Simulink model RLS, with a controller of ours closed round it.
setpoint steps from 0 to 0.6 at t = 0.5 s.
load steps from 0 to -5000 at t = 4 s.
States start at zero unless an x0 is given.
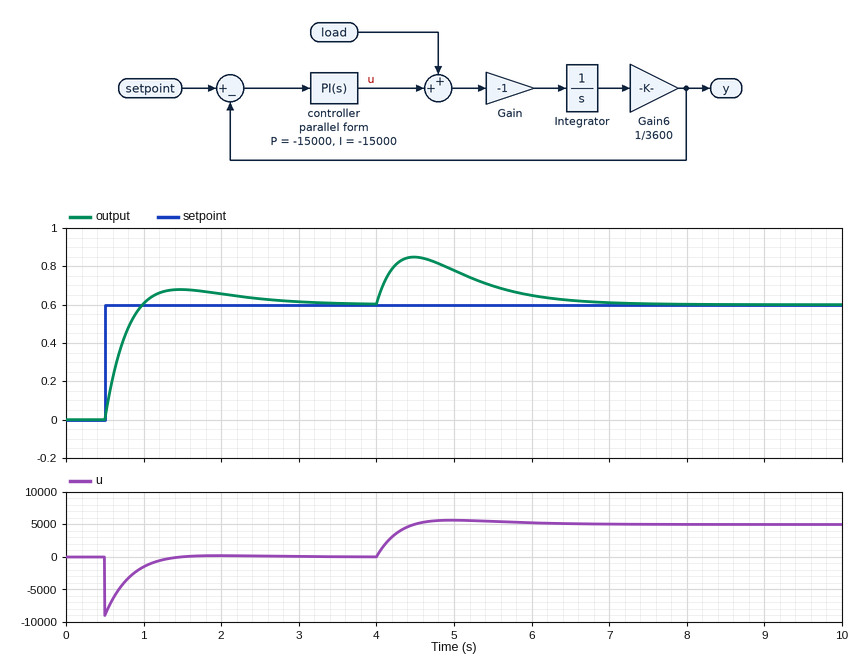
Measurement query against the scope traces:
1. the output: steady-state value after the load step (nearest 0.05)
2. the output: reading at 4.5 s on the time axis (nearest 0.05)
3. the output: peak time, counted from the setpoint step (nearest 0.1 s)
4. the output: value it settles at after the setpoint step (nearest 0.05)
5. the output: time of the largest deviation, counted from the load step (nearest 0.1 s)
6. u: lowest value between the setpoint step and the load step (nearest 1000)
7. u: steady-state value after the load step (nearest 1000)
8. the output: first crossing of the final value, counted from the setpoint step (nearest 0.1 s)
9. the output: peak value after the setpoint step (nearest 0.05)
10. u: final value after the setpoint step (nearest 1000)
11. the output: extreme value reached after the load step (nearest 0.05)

0.60
0.85
1.0 s
0.60
0.5 s
-9000
5000
0.5 s
0.70
0
0.85
